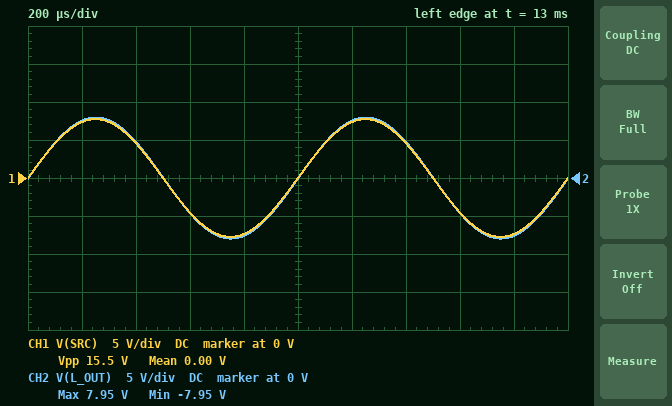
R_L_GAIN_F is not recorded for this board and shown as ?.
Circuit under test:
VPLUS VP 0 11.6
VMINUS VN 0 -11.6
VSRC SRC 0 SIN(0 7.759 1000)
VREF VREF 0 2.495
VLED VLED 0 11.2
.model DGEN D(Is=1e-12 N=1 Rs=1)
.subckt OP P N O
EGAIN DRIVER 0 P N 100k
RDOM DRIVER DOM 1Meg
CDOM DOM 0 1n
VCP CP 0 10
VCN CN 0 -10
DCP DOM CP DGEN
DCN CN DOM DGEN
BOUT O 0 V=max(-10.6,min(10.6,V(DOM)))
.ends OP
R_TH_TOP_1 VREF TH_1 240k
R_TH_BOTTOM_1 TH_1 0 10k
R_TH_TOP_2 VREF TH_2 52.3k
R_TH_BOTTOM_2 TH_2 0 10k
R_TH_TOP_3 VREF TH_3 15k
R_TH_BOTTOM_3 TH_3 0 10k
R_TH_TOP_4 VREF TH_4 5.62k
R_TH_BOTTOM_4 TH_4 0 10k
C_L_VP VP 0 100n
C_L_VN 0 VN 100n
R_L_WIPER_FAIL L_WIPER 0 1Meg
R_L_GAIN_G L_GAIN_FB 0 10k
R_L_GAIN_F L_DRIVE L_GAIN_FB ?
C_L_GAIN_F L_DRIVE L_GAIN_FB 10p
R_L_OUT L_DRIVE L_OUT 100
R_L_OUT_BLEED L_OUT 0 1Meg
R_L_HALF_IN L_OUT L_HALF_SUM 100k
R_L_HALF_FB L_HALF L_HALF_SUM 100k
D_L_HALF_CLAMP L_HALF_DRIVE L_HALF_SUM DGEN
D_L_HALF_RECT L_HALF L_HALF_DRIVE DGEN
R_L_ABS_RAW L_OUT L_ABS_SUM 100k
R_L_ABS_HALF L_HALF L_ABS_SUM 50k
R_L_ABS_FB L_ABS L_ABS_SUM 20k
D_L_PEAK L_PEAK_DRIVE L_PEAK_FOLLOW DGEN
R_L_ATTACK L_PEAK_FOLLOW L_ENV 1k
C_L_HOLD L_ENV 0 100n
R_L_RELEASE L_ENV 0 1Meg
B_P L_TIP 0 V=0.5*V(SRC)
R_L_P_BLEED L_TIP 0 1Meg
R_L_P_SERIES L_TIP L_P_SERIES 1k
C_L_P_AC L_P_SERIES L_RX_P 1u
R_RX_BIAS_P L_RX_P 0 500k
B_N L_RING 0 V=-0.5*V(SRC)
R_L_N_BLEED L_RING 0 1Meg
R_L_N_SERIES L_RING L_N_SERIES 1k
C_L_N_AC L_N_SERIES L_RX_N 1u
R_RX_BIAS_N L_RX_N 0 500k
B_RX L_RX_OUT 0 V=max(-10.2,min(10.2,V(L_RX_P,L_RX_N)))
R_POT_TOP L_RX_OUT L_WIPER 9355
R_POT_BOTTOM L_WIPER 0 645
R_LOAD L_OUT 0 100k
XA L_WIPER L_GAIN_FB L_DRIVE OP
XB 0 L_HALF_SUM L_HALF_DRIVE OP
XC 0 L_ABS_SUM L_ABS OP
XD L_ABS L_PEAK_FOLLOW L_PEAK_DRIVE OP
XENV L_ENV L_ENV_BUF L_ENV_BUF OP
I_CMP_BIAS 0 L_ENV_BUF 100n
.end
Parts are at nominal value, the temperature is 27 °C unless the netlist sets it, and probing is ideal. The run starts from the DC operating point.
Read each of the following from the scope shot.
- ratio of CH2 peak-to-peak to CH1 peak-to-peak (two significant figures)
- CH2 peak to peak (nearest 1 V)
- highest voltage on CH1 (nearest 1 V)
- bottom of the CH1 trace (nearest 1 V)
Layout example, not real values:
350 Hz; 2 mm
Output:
1.0; 16 V; 8 V; -8 V
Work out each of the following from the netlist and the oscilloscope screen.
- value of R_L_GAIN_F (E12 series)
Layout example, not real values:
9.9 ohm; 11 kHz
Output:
150 kΩ
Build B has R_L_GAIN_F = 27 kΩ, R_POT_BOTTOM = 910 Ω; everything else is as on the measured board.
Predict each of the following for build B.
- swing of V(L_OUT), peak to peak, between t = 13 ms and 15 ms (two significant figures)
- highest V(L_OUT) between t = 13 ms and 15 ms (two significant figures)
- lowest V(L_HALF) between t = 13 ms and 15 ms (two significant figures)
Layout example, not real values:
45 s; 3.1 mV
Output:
5.1 V; 2.5 V; -2.5 V
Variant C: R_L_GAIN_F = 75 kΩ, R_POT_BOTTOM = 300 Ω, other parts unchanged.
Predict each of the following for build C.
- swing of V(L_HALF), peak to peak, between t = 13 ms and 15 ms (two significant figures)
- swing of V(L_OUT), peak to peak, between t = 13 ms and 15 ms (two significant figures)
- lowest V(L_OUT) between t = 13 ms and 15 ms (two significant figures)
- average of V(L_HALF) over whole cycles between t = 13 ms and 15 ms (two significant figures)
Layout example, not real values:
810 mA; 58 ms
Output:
2.0 V; 4.1 V; -2.0 V; -650 mV
